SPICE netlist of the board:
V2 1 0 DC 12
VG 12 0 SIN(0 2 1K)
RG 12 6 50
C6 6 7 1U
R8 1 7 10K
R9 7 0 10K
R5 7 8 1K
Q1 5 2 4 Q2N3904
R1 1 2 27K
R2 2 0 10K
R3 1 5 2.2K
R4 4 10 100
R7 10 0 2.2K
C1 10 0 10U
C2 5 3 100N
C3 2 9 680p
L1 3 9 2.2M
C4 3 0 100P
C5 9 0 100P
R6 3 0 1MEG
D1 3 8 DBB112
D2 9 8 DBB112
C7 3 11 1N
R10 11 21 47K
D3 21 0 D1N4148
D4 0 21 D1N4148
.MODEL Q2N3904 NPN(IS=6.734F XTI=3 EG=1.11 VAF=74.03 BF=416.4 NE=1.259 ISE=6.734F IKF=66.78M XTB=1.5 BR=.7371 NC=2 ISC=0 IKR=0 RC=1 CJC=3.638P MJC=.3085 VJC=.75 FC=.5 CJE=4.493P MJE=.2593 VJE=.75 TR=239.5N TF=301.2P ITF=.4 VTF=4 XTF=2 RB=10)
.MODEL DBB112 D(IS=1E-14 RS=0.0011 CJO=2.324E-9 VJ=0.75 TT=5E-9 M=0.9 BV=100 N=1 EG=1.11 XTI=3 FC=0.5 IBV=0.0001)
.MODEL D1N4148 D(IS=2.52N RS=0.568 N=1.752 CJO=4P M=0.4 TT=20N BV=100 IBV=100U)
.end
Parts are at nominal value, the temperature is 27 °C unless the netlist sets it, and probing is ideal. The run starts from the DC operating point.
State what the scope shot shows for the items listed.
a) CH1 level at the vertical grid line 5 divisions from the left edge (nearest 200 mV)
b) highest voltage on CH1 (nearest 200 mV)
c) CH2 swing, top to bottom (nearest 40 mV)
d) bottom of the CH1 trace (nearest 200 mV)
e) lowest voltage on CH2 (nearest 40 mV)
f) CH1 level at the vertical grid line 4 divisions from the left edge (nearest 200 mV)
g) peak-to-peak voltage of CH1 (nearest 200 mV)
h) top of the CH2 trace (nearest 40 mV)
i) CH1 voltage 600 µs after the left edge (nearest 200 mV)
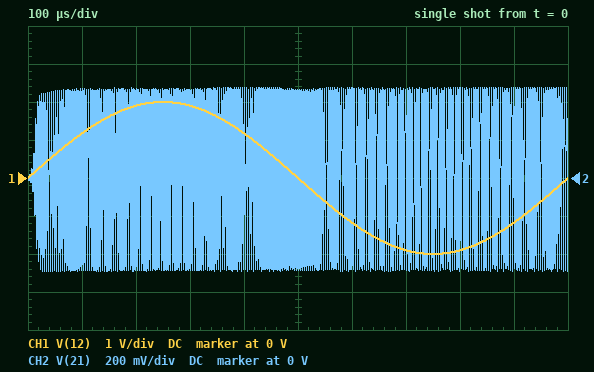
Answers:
0 V
2.0 V
960 mV
-2.0 V
-480 mV
1.2 V
4.0 V
480 mV
-1.2 V
